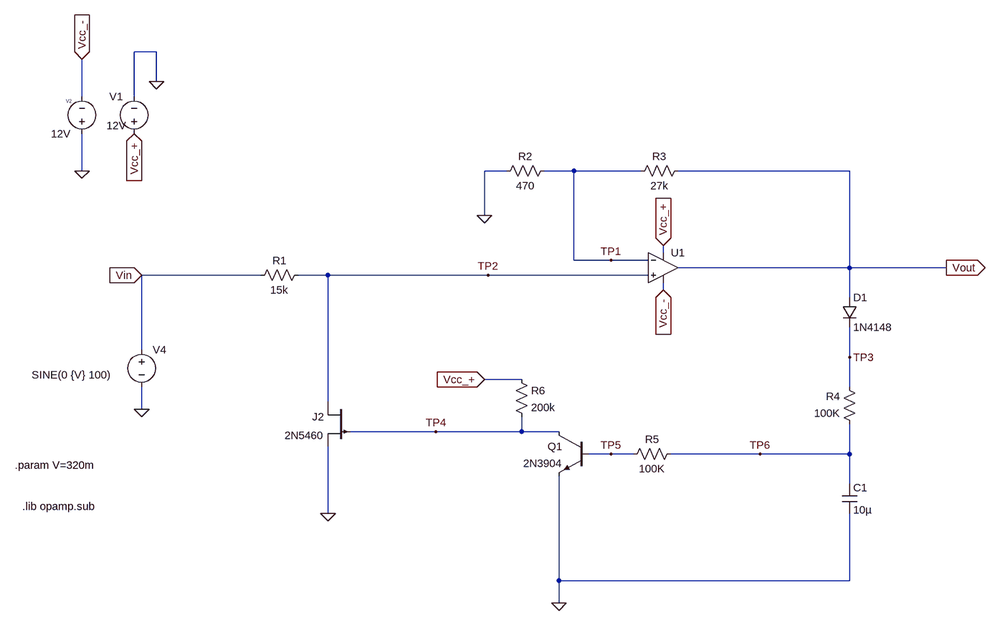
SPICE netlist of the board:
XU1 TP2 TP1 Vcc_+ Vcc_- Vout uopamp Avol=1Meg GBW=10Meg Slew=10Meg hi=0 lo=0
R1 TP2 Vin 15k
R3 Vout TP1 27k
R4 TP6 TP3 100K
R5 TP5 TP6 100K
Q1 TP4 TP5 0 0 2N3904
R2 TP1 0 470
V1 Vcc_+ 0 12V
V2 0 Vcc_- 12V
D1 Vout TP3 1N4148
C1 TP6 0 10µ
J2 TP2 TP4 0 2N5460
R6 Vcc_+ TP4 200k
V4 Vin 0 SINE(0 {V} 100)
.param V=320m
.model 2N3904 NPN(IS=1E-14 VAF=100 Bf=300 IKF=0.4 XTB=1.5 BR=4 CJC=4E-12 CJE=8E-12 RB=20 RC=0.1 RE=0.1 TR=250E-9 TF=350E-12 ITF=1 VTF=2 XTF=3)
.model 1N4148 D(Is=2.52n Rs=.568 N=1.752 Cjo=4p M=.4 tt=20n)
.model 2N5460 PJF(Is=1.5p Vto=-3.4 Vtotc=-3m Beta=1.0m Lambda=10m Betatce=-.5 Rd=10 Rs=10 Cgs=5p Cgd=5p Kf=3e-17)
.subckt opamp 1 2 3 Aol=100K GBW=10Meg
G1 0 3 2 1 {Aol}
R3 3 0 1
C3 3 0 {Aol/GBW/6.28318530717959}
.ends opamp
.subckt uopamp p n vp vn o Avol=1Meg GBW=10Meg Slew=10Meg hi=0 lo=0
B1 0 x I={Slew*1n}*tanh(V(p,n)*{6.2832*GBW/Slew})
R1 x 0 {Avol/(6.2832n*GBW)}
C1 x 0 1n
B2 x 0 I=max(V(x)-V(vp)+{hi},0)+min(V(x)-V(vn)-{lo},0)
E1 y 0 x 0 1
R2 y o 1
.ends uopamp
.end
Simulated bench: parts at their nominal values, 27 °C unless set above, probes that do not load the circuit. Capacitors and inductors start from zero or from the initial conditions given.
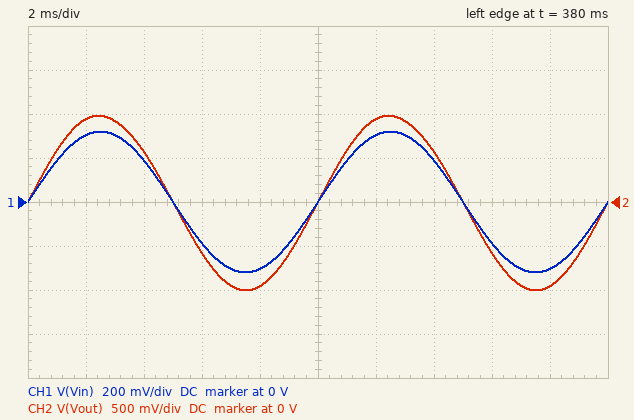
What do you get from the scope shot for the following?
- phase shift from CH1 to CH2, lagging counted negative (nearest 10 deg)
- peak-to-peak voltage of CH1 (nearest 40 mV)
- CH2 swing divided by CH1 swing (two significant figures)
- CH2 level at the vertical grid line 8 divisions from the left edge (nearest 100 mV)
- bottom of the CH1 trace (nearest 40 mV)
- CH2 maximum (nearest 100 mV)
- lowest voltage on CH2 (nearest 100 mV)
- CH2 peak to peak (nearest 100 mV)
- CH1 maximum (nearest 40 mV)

0 deg
640 mV
3.1
-600 mV
-320 mV
1.0 V
-1.0 V
2.0 V
320 mV
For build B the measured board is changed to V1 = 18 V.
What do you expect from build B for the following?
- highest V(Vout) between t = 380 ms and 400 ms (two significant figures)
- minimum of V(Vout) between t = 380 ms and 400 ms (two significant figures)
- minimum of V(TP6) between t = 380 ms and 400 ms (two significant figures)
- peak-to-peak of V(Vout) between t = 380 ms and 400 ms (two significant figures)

1.1 V
-1.1 V
610 mV
2.2 V
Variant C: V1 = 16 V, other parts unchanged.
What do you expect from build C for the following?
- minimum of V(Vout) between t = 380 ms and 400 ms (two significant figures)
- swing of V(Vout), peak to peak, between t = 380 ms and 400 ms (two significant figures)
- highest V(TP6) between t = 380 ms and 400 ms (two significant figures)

-1.1 V
2.1 V
610 mV
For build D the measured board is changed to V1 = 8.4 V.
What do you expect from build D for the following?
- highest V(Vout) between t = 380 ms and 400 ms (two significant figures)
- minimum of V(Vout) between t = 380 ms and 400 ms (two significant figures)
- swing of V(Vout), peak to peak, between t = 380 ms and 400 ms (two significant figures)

910 mV
-930 mV
1.8 V
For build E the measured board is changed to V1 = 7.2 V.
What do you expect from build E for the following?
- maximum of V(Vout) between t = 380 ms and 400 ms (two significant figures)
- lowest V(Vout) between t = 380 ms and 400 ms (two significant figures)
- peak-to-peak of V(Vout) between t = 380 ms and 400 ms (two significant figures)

890 mV
-910 mV
1.8 V
